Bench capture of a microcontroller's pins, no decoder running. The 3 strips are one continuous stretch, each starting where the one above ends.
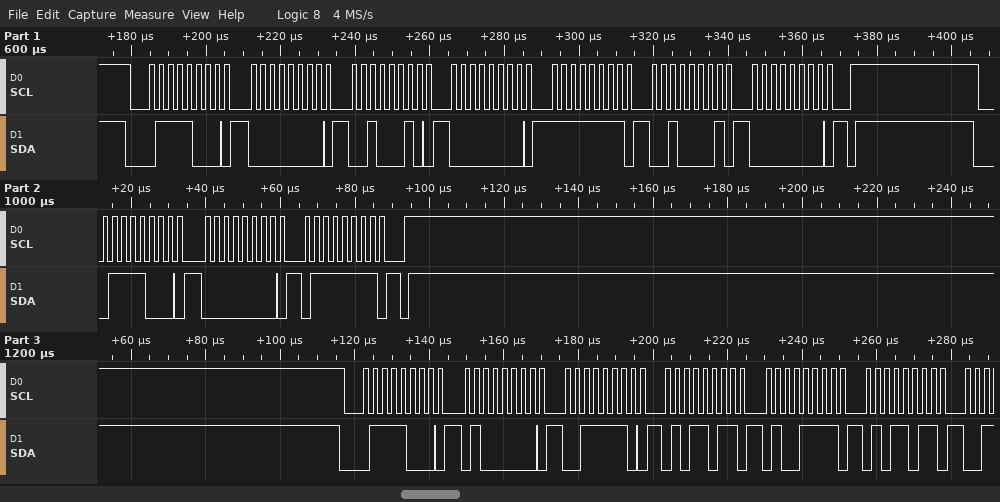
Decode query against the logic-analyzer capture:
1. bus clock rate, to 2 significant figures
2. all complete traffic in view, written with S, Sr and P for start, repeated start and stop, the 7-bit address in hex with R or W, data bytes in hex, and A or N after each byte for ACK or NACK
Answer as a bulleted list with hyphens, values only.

- 400 kHz
- S 3CW A 00 A 22 A 00 A FF A 21 A 00 A P S 3CW A 00 A 7F A P S 3CW A 40 A 3E A 5B A 4F A 5B A
